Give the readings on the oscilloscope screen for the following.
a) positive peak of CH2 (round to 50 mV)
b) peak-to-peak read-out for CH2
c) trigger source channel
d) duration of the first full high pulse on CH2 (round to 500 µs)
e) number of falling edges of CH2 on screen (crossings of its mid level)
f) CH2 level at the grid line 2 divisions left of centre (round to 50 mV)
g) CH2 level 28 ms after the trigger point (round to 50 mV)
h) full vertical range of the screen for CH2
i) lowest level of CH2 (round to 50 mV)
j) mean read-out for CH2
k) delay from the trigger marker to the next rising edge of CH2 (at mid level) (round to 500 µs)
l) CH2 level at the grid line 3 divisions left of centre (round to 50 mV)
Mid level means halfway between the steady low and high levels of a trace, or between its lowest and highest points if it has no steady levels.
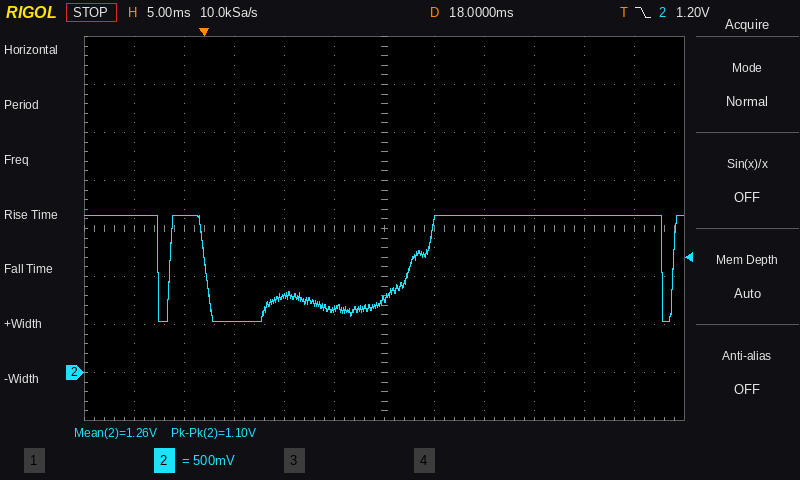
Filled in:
1.65 V
1.10 V
CH2
3.5 ms
3
800 mV
1.65 V
4 V
550 mV
1.26 V
20.5 ms
550 mV
